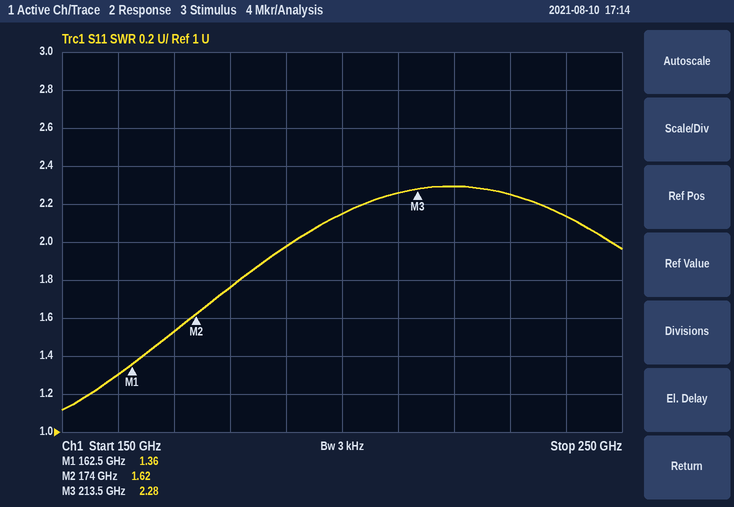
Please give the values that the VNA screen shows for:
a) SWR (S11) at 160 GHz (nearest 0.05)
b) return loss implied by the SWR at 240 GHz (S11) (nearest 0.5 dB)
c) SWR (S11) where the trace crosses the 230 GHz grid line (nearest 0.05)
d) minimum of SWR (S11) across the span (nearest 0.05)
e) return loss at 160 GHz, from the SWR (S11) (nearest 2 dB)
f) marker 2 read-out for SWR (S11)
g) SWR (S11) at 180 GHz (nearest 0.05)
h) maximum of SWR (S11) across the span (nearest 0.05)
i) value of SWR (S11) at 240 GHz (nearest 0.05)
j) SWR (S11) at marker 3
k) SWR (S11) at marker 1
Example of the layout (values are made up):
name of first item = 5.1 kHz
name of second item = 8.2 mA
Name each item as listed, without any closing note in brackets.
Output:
SWR (S11) at 160 GHz = 1.30
return loss implied by the SWR at 240 GHz (S11) = 9.0 dB
SWR (S11) where the trace crosses the 230 GHz grid line = 2.25
minimum of SWR (S11) across the span = 1.10
return loss at 160 GHz, from the SWR (S11) = 18 dB
marker 2 read-out for SWR = 1.62
SWR (S11) at 180 GHz = 1.75
maximum of SWR (S11) across the span = 2.30
value of SWR (S11) at 240 GHz = 2.15
SWR (S11) at marker 3 = 2.28
SWR (S11) at marker 1 = 1.36
